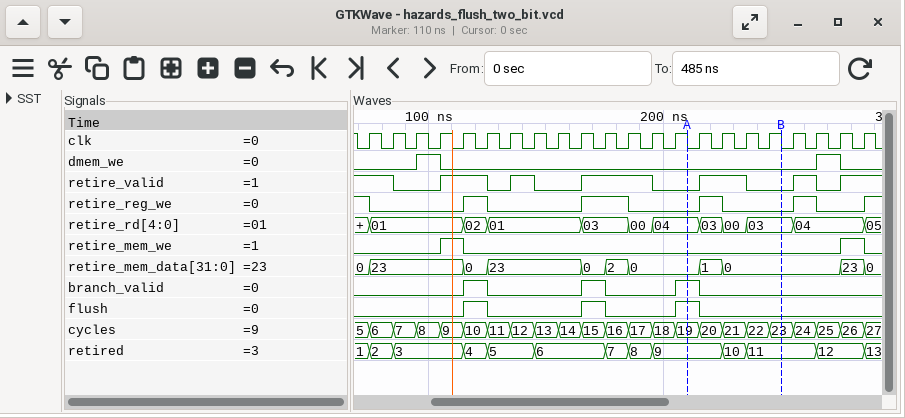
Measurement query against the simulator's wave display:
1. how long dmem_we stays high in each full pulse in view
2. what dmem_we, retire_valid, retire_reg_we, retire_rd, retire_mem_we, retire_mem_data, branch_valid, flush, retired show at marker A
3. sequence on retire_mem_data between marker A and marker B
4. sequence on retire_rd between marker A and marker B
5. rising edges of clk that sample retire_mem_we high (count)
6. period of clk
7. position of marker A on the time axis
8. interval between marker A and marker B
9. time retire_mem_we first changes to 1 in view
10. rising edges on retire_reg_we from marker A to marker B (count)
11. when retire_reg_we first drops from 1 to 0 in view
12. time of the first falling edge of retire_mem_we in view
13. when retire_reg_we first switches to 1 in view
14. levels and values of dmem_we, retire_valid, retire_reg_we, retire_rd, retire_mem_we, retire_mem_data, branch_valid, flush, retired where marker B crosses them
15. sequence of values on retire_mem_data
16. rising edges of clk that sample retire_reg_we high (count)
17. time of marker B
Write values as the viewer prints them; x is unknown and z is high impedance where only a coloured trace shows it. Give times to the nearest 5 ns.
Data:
10 ns, 10 ns
dmem_we=0, retire_valid=0, retire_reg_we=0, retire_rd=04, retire_mem_we=0, retire_mem_data=0, branch_valid=1, flush=1, retired=9
0, 1, 0
04, 03, 00, 03
2
10 ns
210 ns
40 ns
105 ns
1
75 ns
115 ns
115 ns
dmem_we=0, retire_valid=0, retire_reg_we=0, retire_rd=03, retire_mem_we=0, retire_mem_data=0, branch_valid=0, flush=0, retired=11
0, 23, 0, 23, 0, 2, 0, 1, 0, 23, 0
6
250 ns
